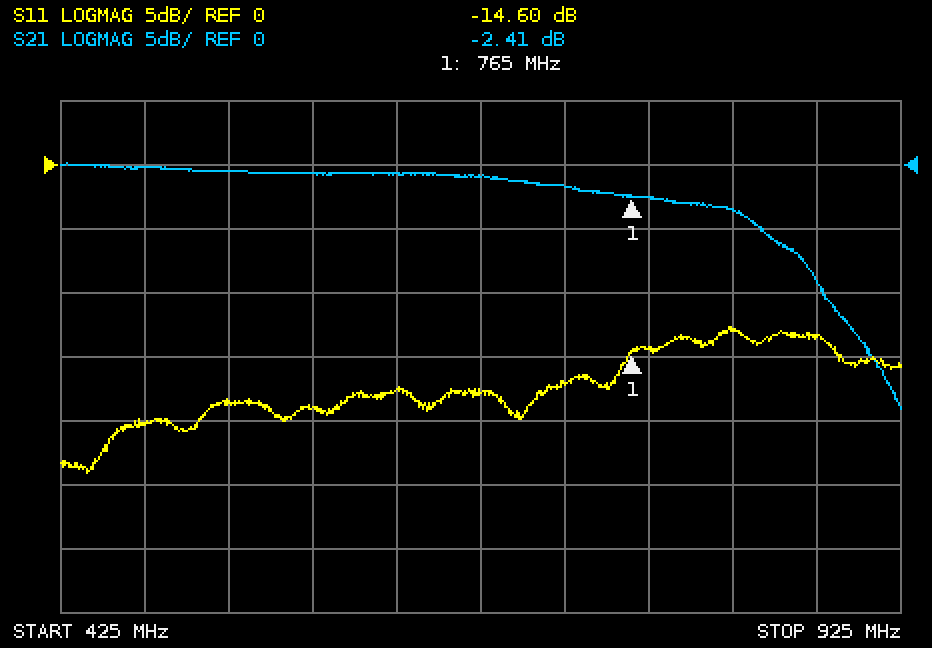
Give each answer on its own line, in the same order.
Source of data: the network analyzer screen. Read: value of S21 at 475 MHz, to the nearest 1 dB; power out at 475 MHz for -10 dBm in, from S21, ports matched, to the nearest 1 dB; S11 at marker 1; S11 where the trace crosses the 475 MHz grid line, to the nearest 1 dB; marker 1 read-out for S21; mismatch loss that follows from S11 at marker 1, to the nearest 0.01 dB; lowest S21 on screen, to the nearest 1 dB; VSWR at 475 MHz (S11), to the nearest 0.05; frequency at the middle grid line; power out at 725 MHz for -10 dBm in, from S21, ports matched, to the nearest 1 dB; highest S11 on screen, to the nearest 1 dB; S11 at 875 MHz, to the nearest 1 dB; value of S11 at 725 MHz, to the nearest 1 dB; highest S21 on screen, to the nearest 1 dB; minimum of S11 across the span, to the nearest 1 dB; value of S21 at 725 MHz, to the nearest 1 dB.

0 dB
-10 dBm
-14.60 dB
-20 dB
-2.41 dB
0.15 dB
-19 dB
1.20
675 MHz
-12 dBm
-13 dB
-13 dB
-17 dB
0 dB
-24 dB
-2 dB
